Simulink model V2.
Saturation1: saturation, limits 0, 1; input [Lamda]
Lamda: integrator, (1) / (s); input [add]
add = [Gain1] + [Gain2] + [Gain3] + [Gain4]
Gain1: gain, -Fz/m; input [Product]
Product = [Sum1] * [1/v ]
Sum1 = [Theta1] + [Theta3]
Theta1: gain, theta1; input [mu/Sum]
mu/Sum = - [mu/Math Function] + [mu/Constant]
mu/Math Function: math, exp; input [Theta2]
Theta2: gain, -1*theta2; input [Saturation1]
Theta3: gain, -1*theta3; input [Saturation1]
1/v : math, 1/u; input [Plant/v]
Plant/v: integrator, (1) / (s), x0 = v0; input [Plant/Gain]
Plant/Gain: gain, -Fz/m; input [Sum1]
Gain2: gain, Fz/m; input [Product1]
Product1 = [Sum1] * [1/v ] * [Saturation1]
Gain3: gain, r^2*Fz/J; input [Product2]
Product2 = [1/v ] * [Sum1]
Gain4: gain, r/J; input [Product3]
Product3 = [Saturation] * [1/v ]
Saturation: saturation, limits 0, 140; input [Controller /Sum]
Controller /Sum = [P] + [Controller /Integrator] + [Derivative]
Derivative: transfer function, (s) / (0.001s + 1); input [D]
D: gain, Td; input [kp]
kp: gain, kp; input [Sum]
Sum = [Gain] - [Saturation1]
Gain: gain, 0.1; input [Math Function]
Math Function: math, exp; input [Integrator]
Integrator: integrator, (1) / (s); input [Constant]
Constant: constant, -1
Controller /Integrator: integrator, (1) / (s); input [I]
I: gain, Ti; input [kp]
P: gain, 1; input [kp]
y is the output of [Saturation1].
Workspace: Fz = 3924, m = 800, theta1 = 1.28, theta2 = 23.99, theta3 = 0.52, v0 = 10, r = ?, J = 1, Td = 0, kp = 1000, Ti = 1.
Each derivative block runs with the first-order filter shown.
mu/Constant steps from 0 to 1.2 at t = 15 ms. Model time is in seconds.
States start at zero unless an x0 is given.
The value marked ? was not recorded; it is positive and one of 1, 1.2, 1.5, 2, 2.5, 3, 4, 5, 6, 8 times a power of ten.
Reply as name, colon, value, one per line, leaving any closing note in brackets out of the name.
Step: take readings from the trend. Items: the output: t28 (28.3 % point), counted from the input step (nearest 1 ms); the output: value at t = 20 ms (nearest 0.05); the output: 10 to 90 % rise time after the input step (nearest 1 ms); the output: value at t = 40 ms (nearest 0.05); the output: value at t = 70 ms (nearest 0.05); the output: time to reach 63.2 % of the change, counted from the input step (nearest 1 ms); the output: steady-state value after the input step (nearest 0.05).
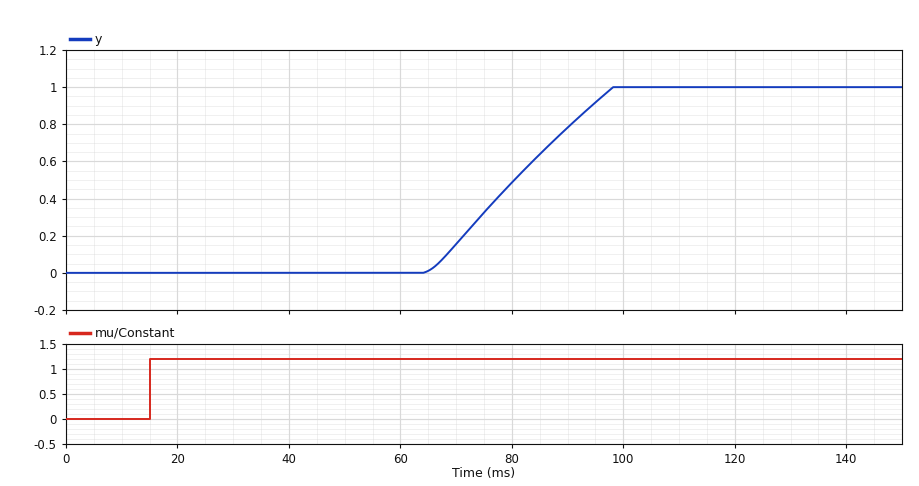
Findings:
the output: t28 (28.3 % point), counted from the input step: 59 ms
the output: value at t = 20 ms: 0.00
the output: 10 to 90 % rise time after the input step: 26 ms
the output: value at t = 40 ms: 0.00
the output: value at t = 70 ms: 0.15
the output: time to reach 63.2 % of the change, counted from the input step: 70 ms
the output: steady-state value after the input step: 1.00
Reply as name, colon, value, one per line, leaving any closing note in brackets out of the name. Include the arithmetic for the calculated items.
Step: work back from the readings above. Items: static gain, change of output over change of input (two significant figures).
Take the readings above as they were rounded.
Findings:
static gain, change of output over change of input: (1 - 0) / (1.2 - 0) = 0.83
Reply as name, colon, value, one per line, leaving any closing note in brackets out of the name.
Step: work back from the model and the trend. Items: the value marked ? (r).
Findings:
the value marked ?: 0.25
